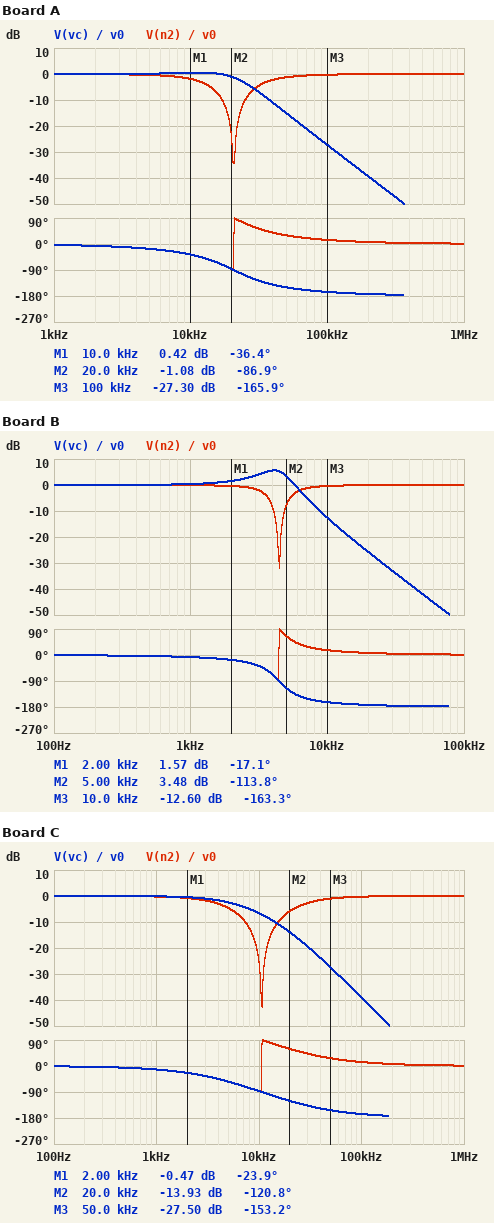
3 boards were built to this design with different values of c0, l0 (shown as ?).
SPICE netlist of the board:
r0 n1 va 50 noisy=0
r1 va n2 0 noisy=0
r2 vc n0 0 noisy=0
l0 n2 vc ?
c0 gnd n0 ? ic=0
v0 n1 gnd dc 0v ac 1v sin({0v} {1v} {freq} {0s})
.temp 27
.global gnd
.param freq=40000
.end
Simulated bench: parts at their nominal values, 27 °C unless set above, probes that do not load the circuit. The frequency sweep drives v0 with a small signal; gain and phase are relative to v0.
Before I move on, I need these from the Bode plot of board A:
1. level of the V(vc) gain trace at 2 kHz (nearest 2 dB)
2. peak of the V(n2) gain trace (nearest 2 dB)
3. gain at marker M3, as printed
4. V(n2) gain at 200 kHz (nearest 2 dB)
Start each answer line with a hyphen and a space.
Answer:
- 0 dB
- 0 dB
- -27.30 dB
- 0 dB
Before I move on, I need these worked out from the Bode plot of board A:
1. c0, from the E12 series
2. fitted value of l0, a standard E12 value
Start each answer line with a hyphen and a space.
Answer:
- 180 nF
- 330 µH
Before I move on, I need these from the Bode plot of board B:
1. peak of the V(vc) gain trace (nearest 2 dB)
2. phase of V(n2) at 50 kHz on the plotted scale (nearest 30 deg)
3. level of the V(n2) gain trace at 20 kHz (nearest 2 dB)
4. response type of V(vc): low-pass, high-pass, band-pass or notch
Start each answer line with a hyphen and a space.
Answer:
- 6 dB
- 0 deg
- 0 dB
- low-pass
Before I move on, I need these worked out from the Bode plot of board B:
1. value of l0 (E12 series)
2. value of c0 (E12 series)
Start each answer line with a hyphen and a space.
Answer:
- 3.3 mH
- 390 nF
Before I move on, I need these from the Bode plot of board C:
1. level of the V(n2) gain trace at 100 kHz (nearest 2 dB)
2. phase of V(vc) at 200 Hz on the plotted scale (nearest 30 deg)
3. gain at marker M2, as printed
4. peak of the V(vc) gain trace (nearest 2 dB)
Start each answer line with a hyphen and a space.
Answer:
- 0 dB
- 0 deg
- -13.93 dB
- 0 dB
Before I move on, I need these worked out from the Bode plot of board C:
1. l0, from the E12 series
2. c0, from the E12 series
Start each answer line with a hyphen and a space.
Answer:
- 330 µH
- 680 nF
